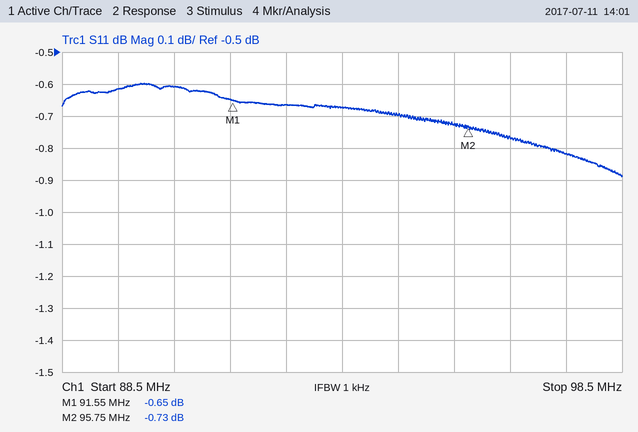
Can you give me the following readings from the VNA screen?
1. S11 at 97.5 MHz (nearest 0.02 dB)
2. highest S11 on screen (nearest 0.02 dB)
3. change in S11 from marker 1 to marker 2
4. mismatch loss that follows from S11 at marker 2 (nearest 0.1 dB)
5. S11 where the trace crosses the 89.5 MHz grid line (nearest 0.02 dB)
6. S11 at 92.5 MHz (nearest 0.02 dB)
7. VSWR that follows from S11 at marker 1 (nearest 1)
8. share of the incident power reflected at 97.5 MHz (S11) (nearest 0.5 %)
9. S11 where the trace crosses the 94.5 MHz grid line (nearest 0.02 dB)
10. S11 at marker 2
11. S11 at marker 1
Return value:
-0.82 dB
-0.60 dB
-0.08 dB
8.1 dB
-0.62 dB
-0.66 dB
27
83.0 %
-0.70 dB
-0.73 dB
-0.65 dB
